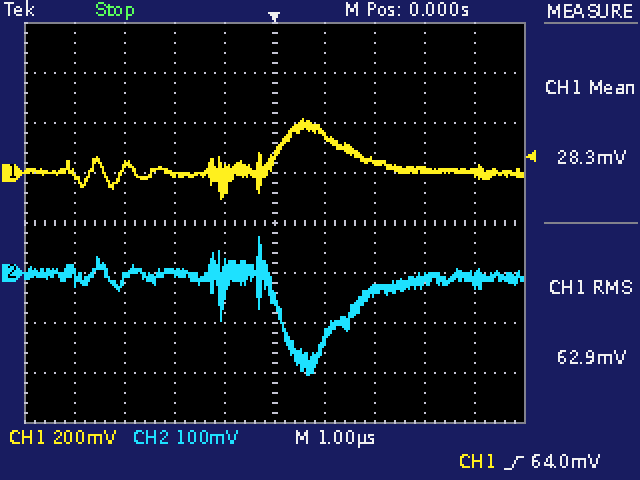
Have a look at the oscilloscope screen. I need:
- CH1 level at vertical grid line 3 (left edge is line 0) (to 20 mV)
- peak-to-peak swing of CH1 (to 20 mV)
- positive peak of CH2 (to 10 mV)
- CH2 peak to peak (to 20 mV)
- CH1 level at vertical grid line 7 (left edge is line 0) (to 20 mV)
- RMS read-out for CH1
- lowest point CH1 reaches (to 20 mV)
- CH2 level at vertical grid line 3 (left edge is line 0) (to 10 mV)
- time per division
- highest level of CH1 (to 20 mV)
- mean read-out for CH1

0 mV
320 mV
70 mV
280 mV
40 mV
62.9 mV
-100 mV
0 mV
1 µs
220 mV
28.3 mV
